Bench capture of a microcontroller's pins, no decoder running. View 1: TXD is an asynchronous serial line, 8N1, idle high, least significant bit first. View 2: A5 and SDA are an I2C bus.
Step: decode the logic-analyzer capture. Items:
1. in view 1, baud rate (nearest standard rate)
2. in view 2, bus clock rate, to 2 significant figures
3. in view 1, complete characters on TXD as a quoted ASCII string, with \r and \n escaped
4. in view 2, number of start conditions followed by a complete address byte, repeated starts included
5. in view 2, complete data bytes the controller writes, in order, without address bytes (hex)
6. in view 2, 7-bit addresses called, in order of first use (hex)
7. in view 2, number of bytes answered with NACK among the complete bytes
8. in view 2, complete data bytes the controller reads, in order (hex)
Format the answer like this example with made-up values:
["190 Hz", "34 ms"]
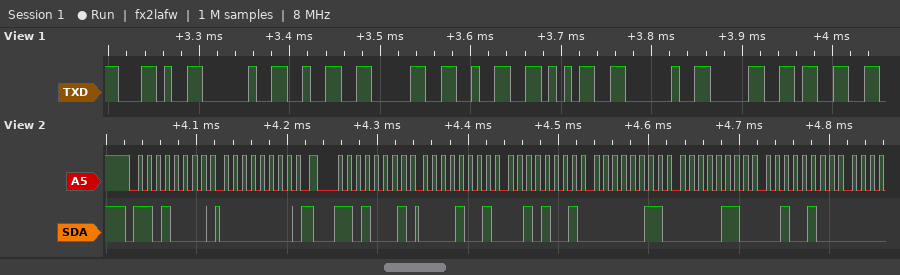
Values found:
["115200 baud", "100 kHz", "\", 2025 03\"", "2", "00", "0x68", "0", "09 29 03 06 24"]
